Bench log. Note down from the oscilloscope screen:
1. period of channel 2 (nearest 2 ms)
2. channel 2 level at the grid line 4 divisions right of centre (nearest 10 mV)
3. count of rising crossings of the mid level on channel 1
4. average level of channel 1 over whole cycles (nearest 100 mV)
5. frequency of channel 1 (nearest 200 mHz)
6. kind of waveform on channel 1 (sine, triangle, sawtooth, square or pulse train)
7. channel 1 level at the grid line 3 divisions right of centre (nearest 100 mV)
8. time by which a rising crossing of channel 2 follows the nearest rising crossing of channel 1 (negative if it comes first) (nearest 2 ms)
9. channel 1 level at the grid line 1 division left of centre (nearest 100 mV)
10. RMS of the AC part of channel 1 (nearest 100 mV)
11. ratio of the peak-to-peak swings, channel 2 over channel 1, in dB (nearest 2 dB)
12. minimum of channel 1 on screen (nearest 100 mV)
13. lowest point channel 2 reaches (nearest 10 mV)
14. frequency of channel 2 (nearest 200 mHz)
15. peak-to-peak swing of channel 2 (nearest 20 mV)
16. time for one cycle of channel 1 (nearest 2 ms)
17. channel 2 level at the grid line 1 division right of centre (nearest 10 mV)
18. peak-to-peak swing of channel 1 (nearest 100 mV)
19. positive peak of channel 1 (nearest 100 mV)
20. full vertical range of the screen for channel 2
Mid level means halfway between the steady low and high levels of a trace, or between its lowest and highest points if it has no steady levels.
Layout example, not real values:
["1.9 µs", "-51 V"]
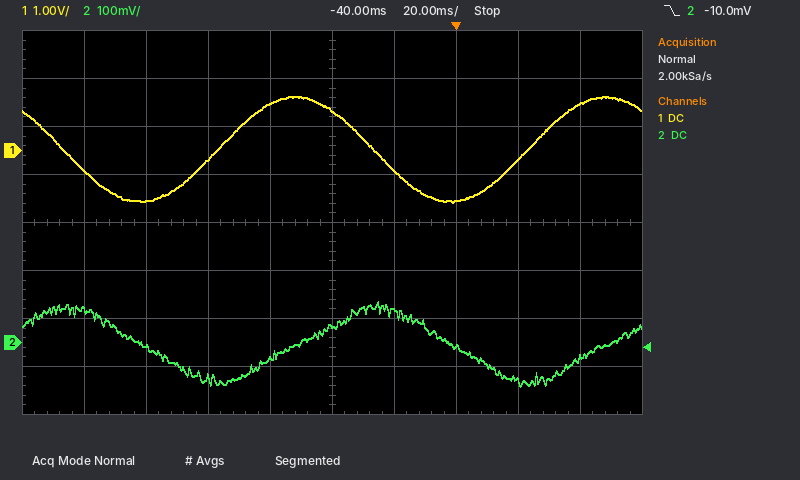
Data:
["100 ms", "-30 mV", "2", "0.0 V", "10.0 Hz", "sine", "-200 mV", "+26 ms", "1.0 V", "800 mV", "-22 dB", "-1.1 V", "-90 mV", "10.0 Hz", "180 mV", "100 ms", "70 mV", "2.2 V", "1.1 V", "800 mV"]
